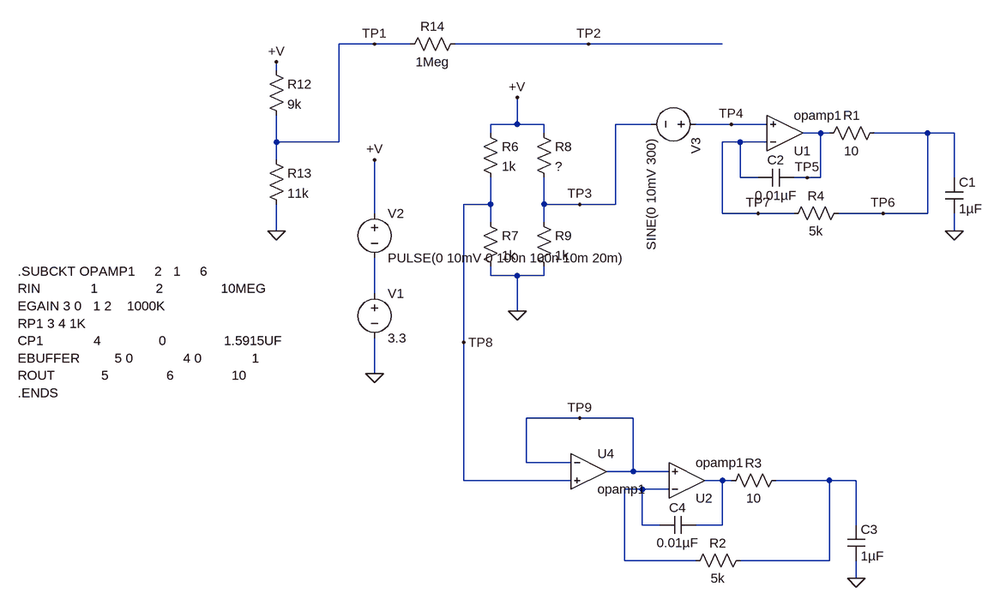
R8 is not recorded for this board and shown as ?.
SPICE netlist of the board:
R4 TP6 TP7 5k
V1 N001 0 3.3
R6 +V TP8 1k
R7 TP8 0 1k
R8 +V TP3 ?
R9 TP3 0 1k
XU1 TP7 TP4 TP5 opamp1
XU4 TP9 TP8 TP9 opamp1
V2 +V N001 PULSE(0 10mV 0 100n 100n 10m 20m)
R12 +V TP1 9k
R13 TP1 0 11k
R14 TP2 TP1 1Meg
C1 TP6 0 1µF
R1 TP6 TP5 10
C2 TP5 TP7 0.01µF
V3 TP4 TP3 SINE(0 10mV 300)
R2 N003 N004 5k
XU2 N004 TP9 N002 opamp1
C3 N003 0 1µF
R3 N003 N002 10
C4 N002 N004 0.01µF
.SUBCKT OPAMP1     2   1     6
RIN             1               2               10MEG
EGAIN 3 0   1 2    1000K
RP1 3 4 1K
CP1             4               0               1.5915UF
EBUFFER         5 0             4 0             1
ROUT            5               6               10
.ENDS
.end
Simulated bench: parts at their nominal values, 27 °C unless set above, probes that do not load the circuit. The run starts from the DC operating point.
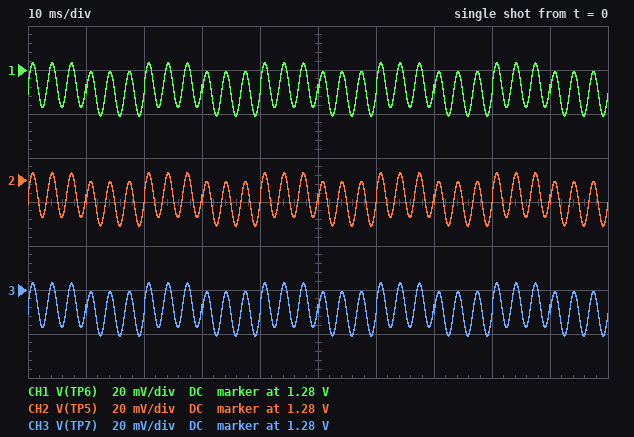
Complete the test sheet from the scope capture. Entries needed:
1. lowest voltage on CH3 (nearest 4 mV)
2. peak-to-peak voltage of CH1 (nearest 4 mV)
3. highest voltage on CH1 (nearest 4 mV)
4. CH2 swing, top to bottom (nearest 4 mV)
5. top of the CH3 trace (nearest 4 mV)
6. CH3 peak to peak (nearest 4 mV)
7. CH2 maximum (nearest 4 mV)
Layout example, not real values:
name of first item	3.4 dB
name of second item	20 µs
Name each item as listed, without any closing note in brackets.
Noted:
lowest voltage on CH3	1.260 V
peak-to-peak voltage of CH1	24 mV
highest voltage on CH1	1.284 V
CH2 swing, top to bottom	24 mV
top of the CH3 trace	1.284 V
CH3 peak to peak	24 mV
CH2 maximum	1.284 V
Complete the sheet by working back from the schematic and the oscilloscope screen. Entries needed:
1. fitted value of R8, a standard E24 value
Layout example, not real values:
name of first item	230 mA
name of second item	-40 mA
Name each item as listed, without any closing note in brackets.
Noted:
fitted value of R8, a standard E24 value	1.6 kΩ
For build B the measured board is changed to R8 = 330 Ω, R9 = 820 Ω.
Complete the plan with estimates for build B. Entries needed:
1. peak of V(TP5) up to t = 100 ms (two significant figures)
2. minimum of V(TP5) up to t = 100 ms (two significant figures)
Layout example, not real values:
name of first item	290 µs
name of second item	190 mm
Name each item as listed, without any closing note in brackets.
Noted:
peak of V(TP5) up to t = 100 ms	2.4 V
minimum of V(TP5) up to t = 100 ms	2.3 V
